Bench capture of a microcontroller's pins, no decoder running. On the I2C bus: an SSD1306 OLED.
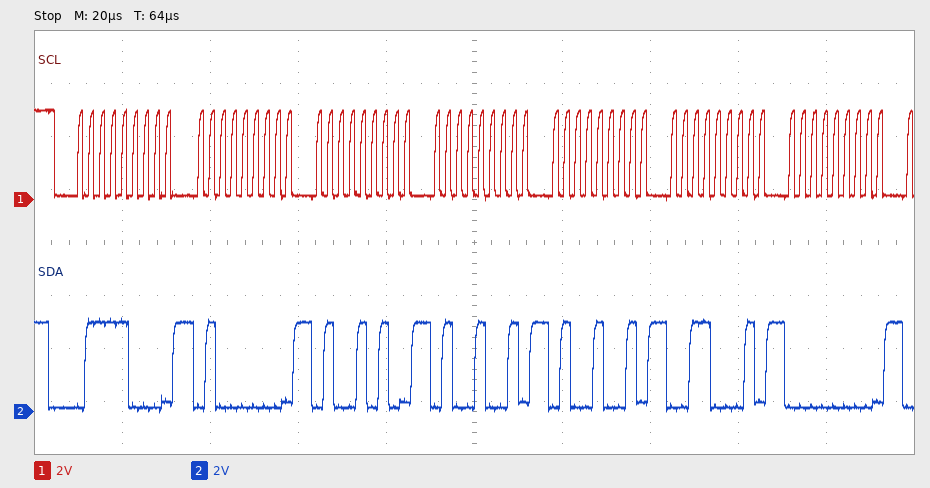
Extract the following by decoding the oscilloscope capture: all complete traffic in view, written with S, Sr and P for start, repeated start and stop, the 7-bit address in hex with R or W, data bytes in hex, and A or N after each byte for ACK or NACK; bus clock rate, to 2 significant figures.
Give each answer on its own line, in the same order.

S 3CW A 40 A 4A A 49 A 49 A 31 A 00 A
400 kHz
